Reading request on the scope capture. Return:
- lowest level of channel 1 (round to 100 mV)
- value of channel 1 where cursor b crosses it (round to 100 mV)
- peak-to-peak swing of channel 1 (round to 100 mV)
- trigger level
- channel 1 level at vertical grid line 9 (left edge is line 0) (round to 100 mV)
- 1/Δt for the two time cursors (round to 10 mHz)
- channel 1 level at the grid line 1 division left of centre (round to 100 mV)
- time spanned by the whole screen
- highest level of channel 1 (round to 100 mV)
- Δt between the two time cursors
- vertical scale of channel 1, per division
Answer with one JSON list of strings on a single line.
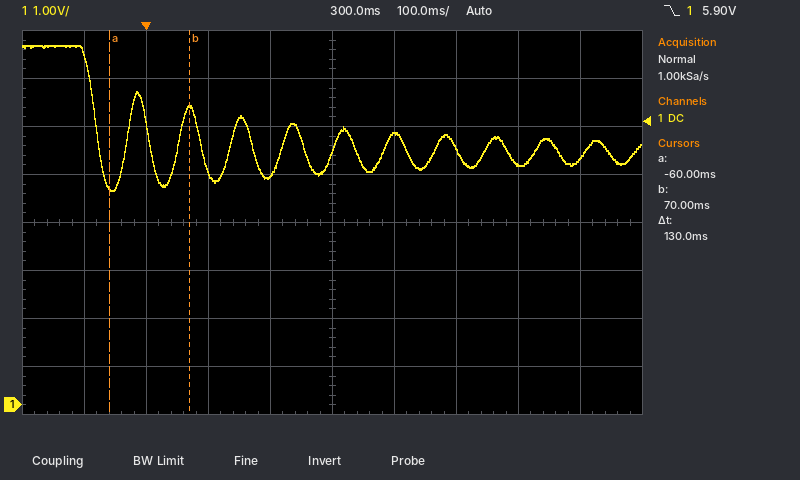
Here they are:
["4.5 V", "6.2 V", "3.0 V", "5.90 V", "5.1 V", "7.69 Hz", "4.8 V", "1 s", "7.5 V", "130 ms", "1 V"]
